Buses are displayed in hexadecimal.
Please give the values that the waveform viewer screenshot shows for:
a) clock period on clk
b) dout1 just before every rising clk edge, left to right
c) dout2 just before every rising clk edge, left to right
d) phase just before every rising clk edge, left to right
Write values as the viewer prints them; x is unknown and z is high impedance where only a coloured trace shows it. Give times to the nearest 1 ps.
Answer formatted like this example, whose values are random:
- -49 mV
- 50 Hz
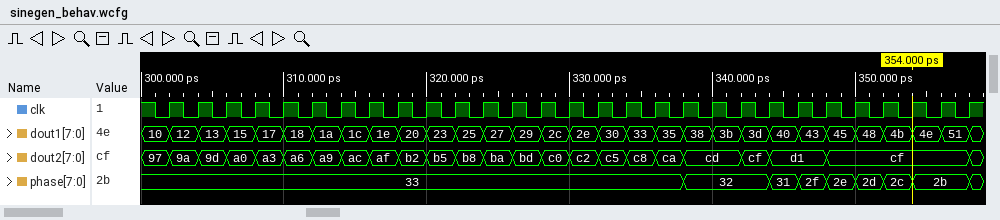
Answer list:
- 2 ps
- 10, 12, 13, 15, 17, 18, 1a, 1c, 1e, 20, 23, 25, 27, 29, 2c, 2e, 30, 33, 35, 38, 3b, 3d, 40, 43, 45, 48, 4b, 4e, 51
- 97, 9a, 9d, a0, a3, a6, a9, ac, af, b2, b5, b8, ba, bd, c0, c2, c5, c8, ca, cd, cd, cf, d1, d1, cf, cf, cf, cf, cf
- 33, 33, 33, 33, 33, 33, 33, 33, 33, 33, 33, 33, 33, 33, 33, 33, 33, 33, 33, 32, 32, 32, 31, 2f, 2e, 2d, 2c, 2b, 2b
